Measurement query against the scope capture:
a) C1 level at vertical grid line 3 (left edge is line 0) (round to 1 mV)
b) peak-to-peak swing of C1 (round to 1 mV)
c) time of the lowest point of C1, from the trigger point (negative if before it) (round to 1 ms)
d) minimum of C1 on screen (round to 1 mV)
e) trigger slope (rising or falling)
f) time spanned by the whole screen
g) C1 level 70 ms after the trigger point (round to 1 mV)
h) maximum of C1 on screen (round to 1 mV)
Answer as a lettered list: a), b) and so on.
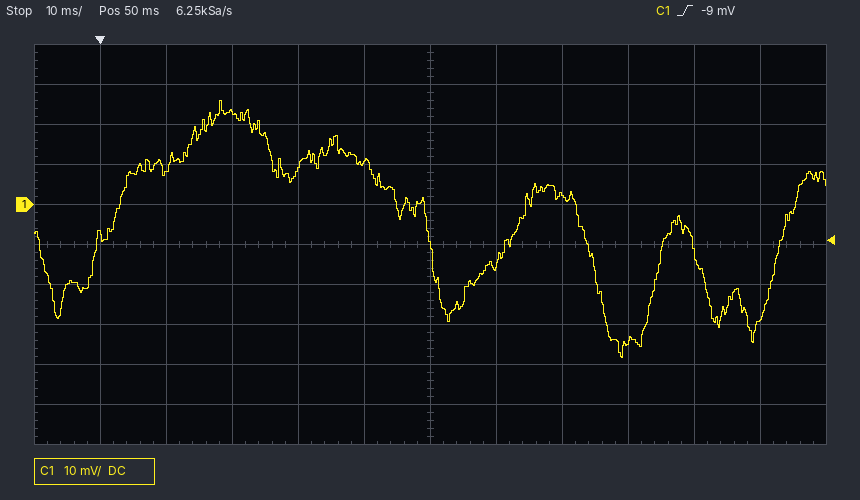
a) 23 mV
b) 64 mV
c) +79 ms
d) -38 mV
e) rising
f) 120 ms
g) 2 mV
h) 26 mV
